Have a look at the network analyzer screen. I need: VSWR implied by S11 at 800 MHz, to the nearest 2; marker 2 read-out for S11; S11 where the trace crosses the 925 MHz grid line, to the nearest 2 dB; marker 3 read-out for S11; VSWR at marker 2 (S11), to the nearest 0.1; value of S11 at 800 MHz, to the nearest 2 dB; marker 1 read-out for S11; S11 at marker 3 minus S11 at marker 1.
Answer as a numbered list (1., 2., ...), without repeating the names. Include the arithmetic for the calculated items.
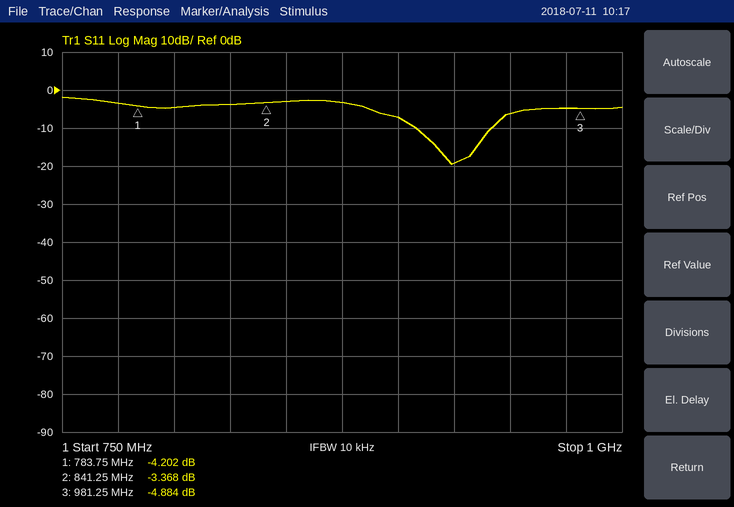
1. |Γ| = 10^(-4/20) = 0.6310; VSWR = (1 + 0.6310)/(1 − 0.6310) ≈ 4
2. -3.368 dB
3. -20 dB
4. -4.884 dB
5. (1 + 0.6786)/(1 − 0.6786) ≈ 5.2
6. -4 dB
7. -4.202 dB
8. -4.884 − (-4.202) = -0.682 dB
